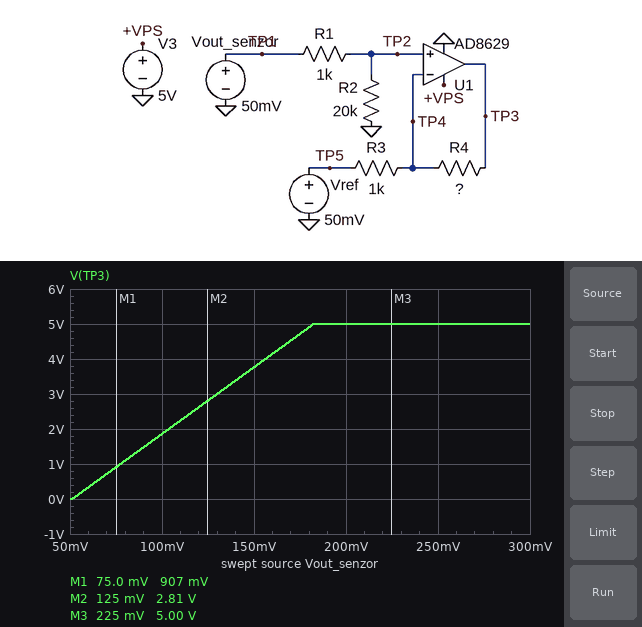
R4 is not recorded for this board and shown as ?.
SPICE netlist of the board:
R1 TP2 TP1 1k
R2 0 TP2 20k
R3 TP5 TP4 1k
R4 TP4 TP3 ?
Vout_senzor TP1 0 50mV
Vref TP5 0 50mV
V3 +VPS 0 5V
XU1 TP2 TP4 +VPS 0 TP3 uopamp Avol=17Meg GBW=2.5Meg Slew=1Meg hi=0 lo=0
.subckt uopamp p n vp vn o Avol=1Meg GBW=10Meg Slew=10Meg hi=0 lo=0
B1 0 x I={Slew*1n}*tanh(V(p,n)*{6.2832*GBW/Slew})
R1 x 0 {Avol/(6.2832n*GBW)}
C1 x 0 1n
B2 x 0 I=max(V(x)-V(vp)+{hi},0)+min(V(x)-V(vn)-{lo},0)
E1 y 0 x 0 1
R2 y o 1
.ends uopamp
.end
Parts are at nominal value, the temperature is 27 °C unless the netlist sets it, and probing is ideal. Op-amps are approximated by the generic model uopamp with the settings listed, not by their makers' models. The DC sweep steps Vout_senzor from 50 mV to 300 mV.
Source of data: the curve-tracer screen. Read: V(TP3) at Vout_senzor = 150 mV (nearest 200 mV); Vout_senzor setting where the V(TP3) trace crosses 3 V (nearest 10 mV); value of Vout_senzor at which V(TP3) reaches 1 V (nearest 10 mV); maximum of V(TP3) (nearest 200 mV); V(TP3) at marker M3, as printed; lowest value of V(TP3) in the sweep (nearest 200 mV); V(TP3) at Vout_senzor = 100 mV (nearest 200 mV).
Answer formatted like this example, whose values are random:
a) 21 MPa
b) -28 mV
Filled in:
a) 3.8 V
b) 130 mV
c) 80 mV
d) 5.0 V
e) 5.00 V
f) 0 V
g) 1.8 V
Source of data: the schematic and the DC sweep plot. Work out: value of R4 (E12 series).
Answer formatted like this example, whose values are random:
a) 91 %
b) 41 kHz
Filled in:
a) 39 kΩ
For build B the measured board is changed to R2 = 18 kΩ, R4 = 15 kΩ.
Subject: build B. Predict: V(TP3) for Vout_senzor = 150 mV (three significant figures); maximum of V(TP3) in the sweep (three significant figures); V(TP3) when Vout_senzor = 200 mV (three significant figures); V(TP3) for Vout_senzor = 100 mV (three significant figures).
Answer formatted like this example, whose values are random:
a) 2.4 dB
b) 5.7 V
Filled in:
a) 1.52 V
b) 3.80 V
c) 2.28 V
d) 766 mV
